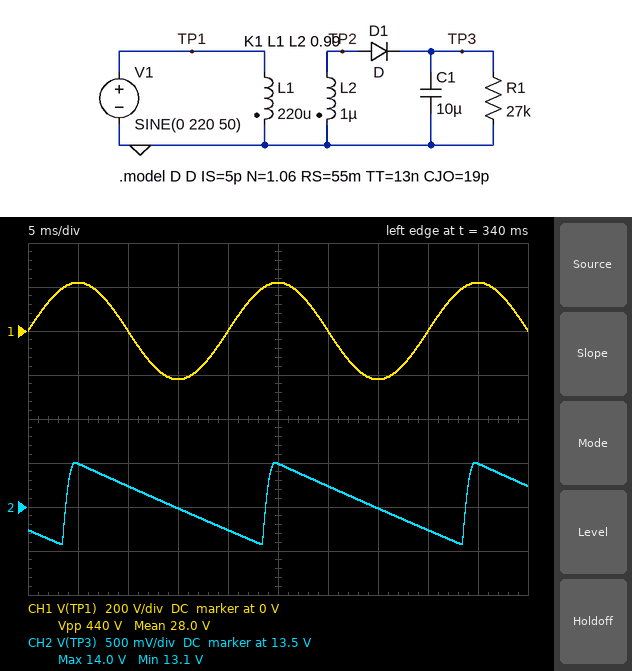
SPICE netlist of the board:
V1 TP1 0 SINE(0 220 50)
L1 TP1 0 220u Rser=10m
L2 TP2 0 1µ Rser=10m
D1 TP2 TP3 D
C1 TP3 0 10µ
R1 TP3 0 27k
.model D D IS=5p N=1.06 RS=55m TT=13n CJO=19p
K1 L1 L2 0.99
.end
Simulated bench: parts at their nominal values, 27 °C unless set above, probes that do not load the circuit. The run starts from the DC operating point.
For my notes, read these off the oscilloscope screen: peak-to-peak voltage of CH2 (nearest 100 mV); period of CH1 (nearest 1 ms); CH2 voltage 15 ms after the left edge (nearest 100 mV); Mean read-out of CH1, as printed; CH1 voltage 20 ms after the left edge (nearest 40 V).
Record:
900 mV
20 ms
13.5 V
28.0 V
0 V
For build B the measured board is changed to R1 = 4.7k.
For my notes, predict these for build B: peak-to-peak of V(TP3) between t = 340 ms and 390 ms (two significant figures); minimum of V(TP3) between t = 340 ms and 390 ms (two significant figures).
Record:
4.3 V
9.7 V
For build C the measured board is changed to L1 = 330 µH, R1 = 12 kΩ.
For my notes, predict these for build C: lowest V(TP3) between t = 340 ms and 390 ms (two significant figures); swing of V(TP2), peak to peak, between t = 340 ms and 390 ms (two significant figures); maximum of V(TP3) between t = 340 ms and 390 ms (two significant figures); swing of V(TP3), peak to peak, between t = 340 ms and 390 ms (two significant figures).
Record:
9.8 V
24 V
11 V
1.6 V
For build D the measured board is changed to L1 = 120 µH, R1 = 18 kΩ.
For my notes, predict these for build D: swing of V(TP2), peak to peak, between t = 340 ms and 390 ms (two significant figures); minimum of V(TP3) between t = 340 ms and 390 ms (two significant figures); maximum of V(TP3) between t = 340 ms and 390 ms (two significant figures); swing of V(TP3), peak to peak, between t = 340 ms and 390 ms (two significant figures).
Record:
38 V
17 V
19 V
1.8 V
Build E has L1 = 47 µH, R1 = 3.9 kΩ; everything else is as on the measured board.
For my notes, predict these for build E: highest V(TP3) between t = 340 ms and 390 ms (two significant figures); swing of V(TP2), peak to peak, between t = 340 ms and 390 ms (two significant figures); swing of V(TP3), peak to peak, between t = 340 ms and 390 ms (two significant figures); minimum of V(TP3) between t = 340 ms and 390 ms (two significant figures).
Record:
26 V
53 V
9.1 V
17 V
